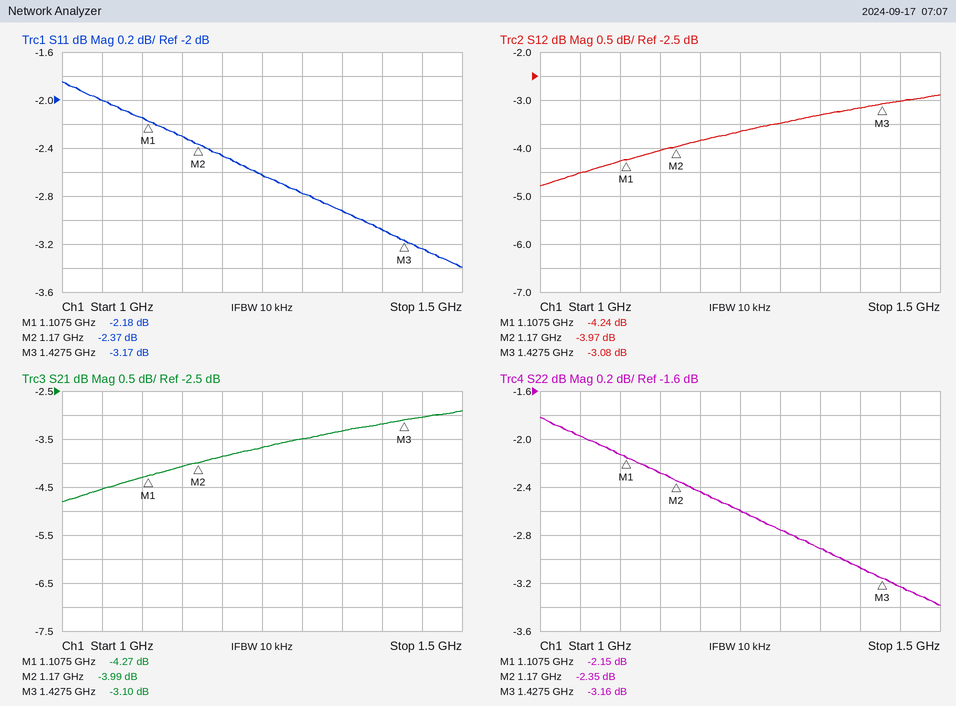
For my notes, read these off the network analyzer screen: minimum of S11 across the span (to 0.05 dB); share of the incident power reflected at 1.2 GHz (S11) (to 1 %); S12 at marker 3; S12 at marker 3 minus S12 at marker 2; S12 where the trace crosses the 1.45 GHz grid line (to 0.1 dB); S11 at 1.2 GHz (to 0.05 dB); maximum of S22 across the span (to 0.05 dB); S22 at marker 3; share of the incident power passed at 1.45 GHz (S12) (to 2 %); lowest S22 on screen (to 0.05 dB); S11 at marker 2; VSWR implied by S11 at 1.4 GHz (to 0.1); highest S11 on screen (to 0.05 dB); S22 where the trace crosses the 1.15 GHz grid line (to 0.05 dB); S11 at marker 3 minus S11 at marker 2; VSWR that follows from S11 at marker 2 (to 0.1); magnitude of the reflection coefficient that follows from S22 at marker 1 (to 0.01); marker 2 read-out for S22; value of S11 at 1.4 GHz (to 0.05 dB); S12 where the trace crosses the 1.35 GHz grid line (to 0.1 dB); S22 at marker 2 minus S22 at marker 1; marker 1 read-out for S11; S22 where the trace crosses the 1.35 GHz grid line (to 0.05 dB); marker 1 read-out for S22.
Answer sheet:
-3.40 dB
57 %
-3.08 dB
0.89 dB
-3.0 dB
-2.45 dB
-1.80 dB
-3.16 dB
50 %
-3.40 dB
-2.37 dB
5.7
-1.85 dB
-2.30 dB
-0.80 dB
7.4
0.78
-2.35 dB
-3.10 dB
-3.3 dB
-0.20 dB
-2.18 dB
-2.90 dB
-2.15 dB
